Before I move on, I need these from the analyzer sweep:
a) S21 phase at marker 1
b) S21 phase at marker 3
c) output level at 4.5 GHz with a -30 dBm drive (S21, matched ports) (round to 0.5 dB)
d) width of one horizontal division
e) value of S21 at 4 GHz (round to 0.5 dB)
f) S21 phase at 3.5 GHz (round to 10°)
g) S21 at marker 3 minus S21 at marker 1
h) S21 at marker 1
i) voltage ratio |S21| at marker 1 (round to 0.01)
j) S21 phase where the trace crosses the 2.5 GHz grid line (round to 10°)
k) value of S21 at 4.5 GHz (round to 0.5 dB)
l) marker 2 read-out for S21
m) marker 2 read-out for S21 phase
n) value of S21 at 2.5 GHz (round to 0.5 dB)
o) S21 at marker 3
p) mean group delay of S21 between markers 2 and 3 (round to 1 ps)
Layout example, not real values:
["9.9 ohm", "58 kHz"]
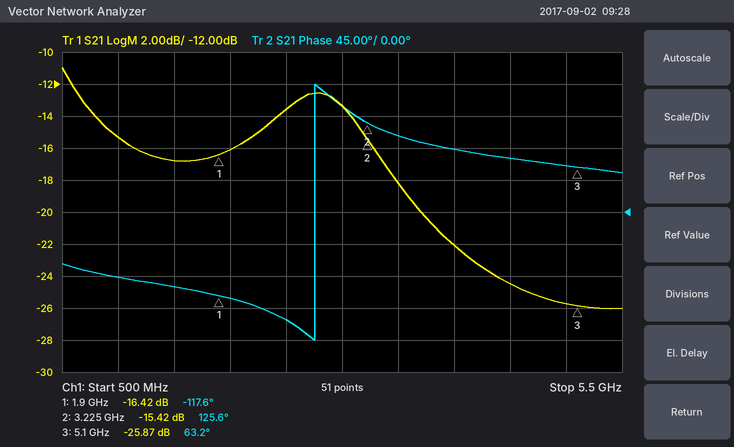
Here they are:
["-117.6°", "63.2°", "-54.5 dBm", "500 MHz", "-22.0 dB", "110°", "-9.45 dB", "-16.42 dB", "0.15", "-150°", "-24.5 dB", "-15.42 dB", "125.6°", "-13.5 dB", "-25.87 dB", "92 ps"]
